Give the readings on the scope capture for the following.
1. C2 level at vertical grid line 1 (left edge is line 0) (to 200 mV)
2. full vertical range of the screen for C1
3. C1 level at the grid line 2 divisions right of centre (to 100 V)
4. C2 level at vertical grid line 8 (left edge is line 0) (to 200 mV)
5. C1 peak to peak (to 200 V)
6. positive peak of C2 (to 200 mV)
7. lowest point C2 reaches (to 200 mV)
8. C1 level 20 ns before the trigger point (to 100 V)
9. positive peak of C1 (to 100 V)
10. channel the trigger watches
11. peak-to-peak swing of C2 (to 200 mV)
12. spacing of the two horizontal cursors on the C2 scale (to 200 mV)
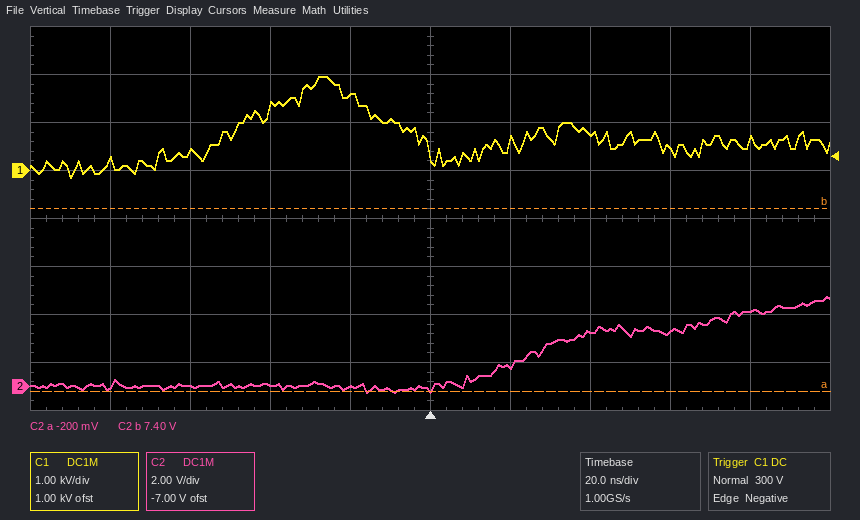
0.0 V
8 kV
800 V
2.2 V
2.2 kV
3.8 V
-200 mV
1.6 kV
2.0 kV
C1
4.0 V
7.6 V
